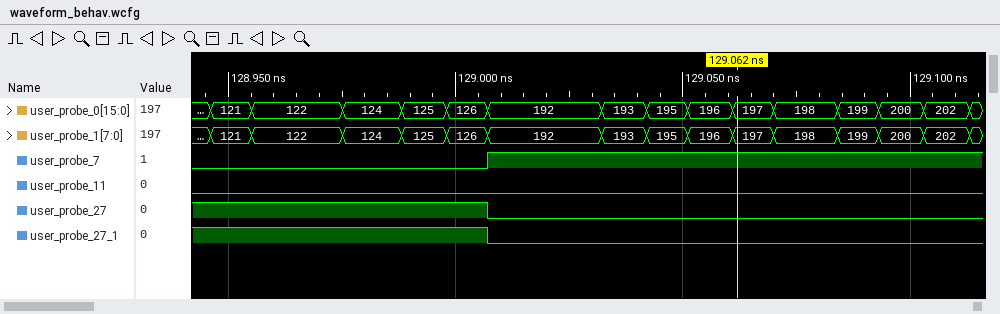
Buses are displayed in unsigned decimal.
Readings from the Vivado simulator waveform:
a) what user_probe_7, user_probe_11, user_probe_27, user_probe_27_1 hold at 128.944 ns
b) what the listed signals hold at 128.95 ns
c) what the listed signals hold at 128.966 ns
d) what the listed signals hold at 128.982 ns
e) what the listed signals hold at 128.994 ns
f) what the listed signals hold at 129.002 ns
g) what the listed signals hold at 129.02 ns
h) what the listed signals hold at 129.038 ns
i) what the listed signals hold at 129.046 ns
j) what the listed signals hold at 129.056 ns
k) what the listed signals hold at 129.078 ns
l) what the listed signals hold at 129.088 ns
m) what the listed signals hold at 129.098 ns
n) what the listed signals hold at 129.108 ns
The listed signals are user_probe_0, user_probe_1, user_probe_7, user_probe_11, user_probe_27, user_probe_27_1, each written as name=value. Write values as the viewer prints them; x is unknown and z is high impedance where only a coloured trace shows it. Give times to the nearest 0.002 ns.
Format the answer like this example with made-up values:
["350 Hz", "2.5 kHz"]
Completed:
["user_probe_7=0, user_probe_11=0, user_probe_27=1, user_probe_27_1=1", "user_probe_0=121, user_probe_1=121, user_probe_7=0, user_probe_11=0, user_probe_27=1, user_probe_27_1=1", "user_probe_0=122, user_probe_1=122, user_probe_7=0, user_probe_11=0, user_probe_27=1, user_probe_27_1=1", "user_probe_0=124, user_probe_1=124, user_probe_7=0, user_probe_11=0, user_probe_27=1, user_probe_27_1=1", "user_probe_0=125, user_probe_1=125, user_probe_7=0, user_probe_11=0, user_probe_27=1, user_probe_27_1=1", "user_probe_0=126, user_probe_1=126, user_probe_7=0, user_probe_11=0, user_probe_27=1, user_probe_27_1=1", "user_probe_0=192, user_probe_1=192, user_probe_7=1, user_probe_11=0, user_probe_27=0, user_probe_27_1=0", "user_probe_0=193, user_probe_1=193, user_probe_7=1, user_probe_11=0, user_probe_27=0, user_probe_27_1=0", "user_probe_0=195, user_probe_1=195, user_probe_7=1, user_probe_11=0, user_probe_27=0, user_probe_27_1=0", "user_probe_0=196, user_probe_1=196, user_probe_7=1, user_probe_11=0, user_probe_27=0, user_probe_27_1=0", "user_probe_0=198, user_probe_1=198, user_probe_7=1, user_probe_11=0, user_probe_27=0, user_probe_27_1=0", "user_probe_0=199, user_probe_1=199, user_probe_7=1, user_probe_11=0, user_probe_27=0, user_probe_27_1=0", "user_probe_0=200, user_probe_1=200, user_probe_7=1, user_probe_11=0, user_probe_27=0, user_probe_27_1=0", "user_probe_0=202, user_probe_1=202, user_probe_7=1, user_probe_11=0, user_probe_27=0, user_probe_27_1=0"]
